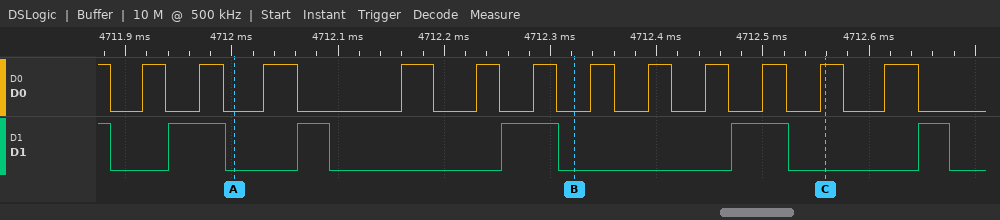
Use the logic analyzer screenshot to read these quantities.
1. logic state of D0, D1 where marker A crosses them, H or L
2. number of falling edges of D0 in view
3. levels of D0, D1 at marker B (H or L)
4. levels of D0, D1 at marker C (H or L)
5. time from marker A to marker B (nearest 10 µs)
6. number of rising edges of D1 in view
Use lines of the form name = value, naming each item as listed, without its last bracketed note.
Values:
logic state of D0, D1 where marker A crosses them, H or L = D0=L, D1=L
number of falling edges of D0 in view = 13
levels of D0, D1 at marker B = D0=L, D1=L
levels of D0, D1 at marker C = D0=H, D1=L
time from marker A to marker B = 320 µs
number of rising edges of D1 in view = 5
